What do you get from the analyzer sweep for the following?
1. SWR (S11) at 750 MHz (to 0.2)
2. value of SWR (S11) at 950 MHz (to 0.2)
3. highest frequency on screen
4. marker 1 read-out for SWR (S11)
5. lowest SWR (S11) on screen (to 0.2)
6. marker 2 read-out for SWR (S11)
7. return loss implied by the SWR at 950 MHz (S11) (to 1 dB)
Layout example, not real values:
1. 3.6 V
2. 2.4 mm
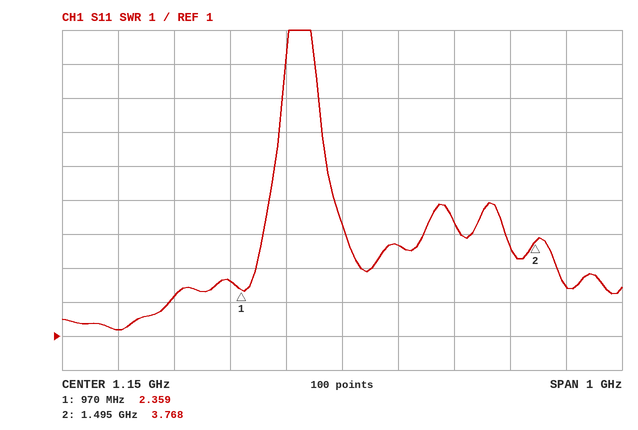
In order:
1. 1.2
2. 2.6
3. 1.65 GHz
4. 2.359
5. 1.2
6. 3.768
7. 7 dB
